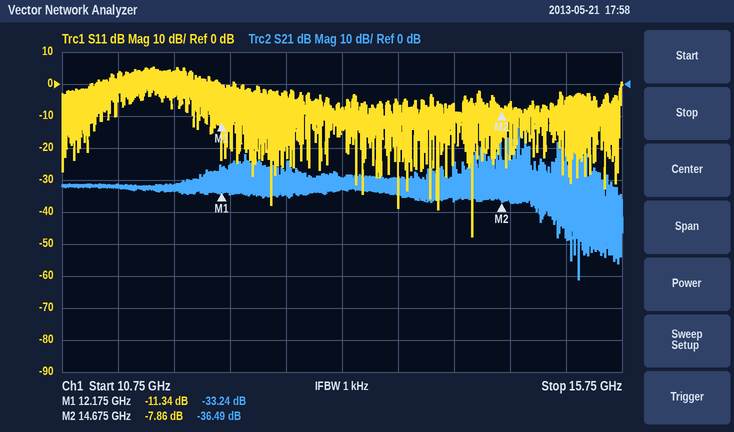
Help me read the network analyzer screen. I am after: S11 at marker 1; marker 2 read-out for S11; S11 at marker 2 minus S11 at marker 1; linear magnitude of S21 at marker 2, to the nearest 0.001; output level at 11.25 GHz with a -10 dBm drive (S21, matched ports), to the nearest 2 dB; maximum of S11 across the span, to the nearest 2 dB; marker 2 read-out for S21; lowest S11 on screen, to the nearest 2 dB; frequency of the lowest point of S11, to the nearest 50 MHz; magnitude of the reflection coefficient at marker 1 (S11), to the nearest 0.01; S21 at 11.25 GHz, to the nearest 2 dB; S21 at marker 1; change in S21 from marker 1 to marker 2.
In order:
-11.34 dB
-7.86 dB
3.48 dB
0.015
-42 dBm
6 dB
-36.49 dB
-48 dB
14.40 GHz
0.27
-32 dB
-33.24 dB
-3.25 dB
